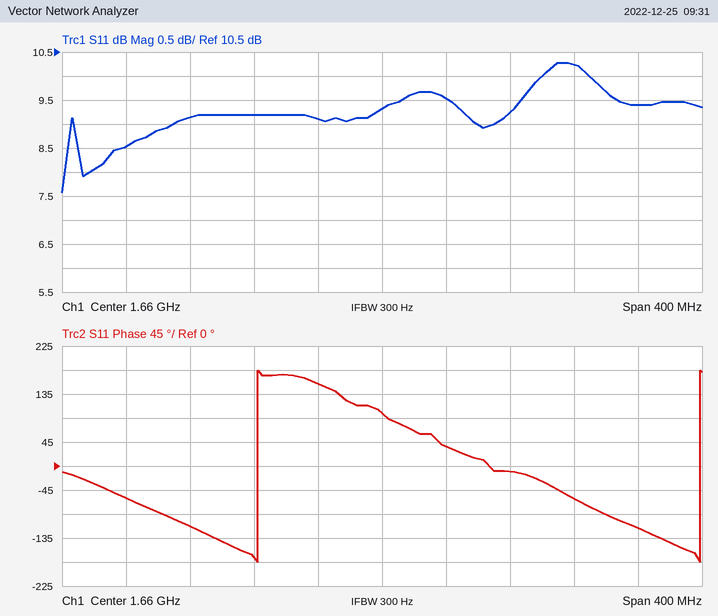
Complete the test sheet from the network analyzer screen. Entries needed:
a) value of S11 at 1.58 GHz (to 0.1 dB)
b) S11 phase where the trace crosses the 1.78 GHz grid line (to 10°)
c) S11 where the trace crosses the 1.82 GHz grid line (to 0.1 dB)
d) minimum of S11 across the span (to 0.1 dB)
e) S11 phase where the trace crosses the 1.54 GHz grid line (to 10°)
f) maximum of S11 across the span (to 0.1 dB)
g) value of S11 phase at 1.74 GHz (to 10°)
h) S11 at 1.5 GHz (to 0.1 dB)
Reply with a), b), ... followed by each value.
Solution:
a) 9.2 dB
b) -60°
c) 9.4 dB
d) 7.6 dB
e) -110°
f) 10.3 dB
g) -10°
h) 8.5 dB
